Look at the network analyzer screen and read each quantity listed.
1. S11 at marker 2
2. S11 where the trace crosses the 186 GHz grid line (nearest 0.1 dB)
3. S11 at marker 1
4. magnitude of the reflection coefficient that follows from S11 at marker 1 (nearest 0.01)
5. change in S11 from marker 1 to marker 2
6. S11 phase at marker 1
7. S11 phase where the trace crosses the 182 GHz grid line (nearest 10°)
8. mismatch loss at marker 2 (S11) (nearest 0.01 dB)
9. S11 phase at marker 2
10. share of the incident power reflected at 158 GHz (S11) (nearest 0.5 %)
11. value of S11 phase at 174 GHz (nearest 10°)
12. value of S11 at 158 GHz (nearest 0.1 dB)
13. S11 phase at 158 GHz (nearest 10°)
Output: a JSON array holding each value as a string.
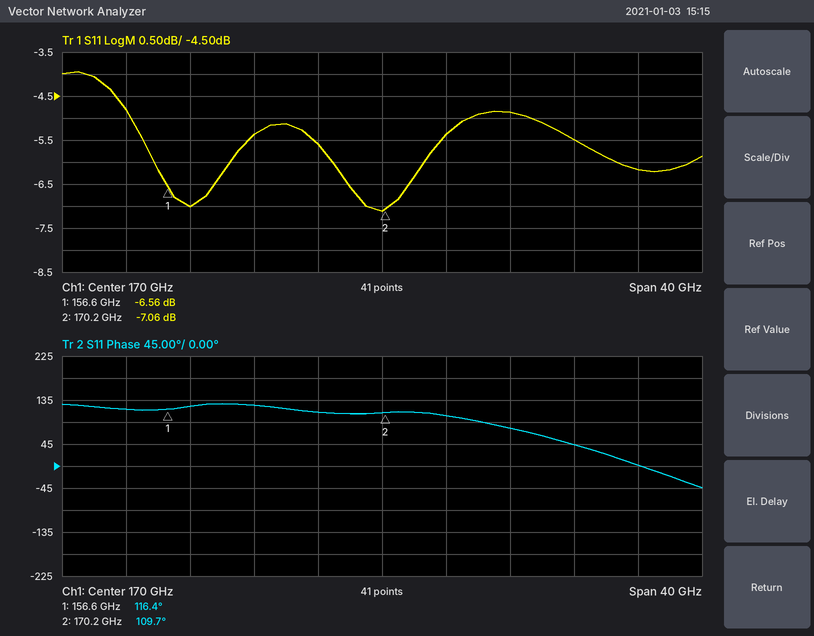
["-7.06 dB", "-6.2 dB", "-6.56 dB", "0.47", "-0.50 dB", "116.4°", "40°", "0.95 dB", "109.7°", "20.0 %", "100°", "-7.0 dB", "120°"]
